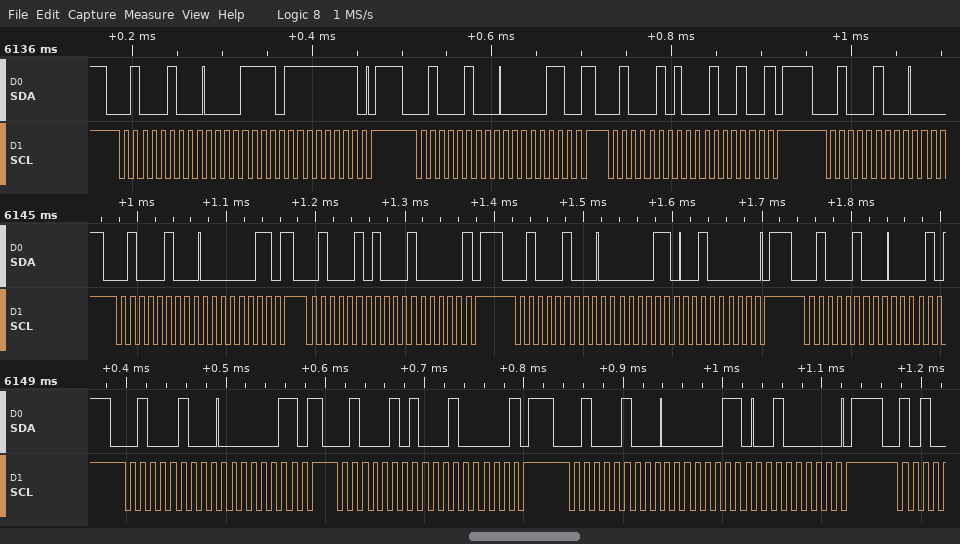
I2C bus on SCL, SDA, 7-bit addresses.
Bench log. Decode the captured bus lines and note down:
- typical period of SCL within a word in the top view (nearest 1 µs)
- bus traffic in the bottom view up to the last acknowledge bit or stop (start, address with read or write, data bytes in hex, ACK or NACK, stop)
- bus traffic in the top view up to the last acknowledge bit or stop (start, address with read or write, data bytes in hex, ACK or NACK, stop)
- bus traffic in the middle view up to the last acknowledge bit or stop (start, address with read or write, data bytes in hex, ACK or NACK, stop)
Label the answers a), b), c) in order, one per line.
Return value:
a) 10 µs
b) start, address 22 write ACK, 03 ACK, repeated start, address 22 read ACK, 20 NACK, stop, start, address 22 write ACK, 03 ACK, 20 ACK, stop
c) start, address 22 write ACK, 0F ACK, FF ACK, stop, start, address 22 write ACK, 06 ACK, repeated start, address 22 read ACK, 24 NACK, stop, start, address 22 write ACK
d) start, address 22 write ACK, 03 ACK, repeated start, address 22 read ACK, 20 NACK, stop, start, address 22 write ACK, 03 ACK, 20 ACK, stop, start, address 22 write ACK
